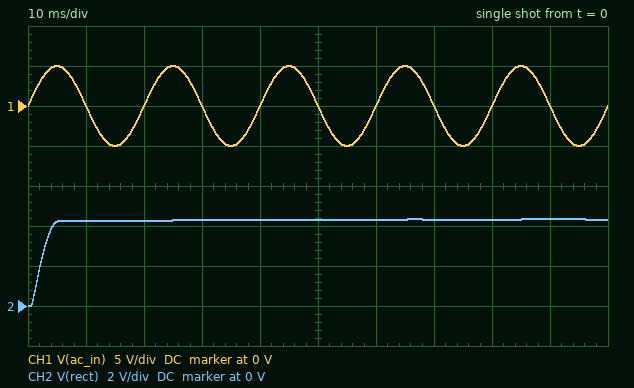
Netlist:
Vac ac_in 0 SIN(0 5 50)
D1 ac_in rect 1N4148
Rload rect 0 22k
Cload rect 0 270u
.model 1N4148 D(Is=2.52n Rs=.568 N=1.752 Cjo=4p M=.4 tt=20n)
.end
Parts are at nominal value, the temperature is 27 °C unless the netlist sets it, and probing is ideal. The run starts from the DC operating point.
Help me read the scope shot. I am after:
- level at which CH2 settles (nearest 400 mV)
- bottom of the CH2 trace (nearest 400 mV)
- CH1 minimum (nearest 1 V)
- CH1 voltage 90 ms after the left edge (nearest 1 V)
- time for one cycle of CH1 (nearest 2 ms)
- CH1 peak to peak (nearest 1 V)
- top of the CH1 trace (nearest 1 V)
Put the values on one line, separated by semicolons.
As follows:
4.4 V; 0 V; -5 V; 0 V; 20 ms; 10 V; 5 V
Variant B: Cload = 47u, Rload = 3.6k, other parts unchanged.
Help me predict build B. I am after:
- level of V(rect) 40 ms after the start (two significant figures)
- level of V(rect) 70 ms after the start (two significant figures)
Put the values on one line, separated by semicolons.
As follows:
4.0 V; 4.2 V
